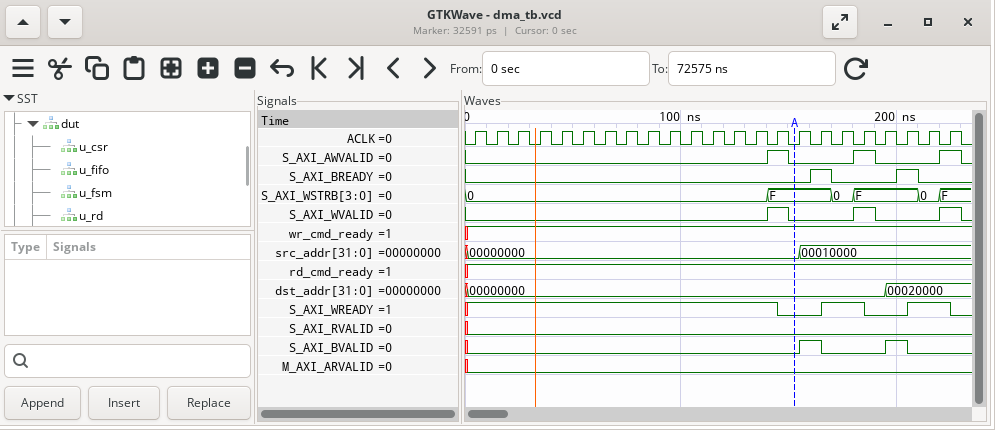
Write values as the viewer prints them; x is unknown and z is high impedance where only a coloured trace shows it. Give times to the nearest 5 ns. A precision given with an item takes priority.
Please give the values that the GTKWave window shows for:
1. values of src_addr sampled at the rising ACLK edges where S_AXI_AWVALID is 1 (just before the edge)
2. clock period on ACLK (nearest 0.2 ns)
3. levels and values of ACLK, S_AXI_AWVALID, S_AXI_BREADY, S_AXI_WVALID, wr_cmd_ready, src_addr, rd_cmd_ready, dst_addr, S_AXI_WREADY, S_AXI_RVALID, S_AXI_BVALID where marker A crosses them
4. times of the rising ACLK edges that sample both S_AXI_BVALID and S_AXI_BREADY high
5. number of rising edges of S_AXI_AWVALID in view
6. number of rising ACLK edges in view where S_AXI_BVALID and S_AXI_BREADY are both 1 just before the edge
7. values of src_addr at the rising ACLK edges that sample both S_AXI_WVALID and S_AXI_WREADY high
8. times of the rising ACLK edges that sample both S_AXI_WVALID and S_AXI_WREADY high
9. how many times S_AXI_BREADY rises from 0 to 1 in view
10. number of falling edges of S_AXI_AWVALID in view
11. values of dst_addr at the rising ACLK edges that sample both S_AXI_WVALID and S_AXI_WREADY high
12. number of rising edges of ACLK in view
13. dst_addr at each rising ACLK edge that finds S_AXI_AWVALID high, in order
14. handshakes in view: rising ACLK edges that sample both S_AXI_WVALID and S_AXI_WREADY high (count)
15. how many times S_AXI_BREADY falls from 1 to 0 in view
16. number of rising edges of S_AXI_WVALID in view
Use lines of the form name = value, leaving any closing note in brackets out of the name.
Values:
values of src_addr sampled at the rising ACLK edges where S_AXI_AWVALID is 1 = 00000000, 00010000, 00010000
clock period on ACLK = 10 ns
levels and values of ACLK, S_AXI_AWVALID, S_AXI_BREADY, S_AXI_WVALID, wr_cmd_ready, src_addr, rd_cmd_ready, dst_addr, S_AXI_WREADY, S_AXI_RVALID, S_AXI_BVALID where marker A crosses them = ACLK=0, S_AXI_AWVALID=0, S_AXI_BREADY=0, S_AXI_WVALID=0, wr_cmd_ready=1, src_addr=00000000, rd_cmd_ready=1, dst_addr=00000000, S_AXI_WREADY=0, S_AXI_RVALID=0, S_AXI_BVALID=0
times of the rising ACLK edges that sample both S_AXI_BVALID and S_AXI_BREADY high = 165 ns, 205 ns
number of rising edges of S_AXI_AWVALID in view = 3
number of rising ACLK edges in view where S_AXI_BVALID and S_AXI_BREADY are both 1 just before the edge = 2
values of src_addr at the rising ACLK edges that sample both S_AXI_WVALID and S_AXI_WREADY high = 00000000, 00010000, 00010000
times of the rising ACLK edges that sample both S_AXI_WVALID and S_AXI_WREADY high = 145 ns, 185 ns, 225 ns
how many times S_AXI_BREADY rises from 0 to 1 in view = 2
number of falling edges of S_AXI_AWVALID in view = 3
values of dst_addr at the rising ACLK edges that sample both S_AXI_WVALID and S_AXI_WREADY high = 00000000, 00000000, 00020000
number of rising edges of ACLK in view = 23
dst_addr at each rising ACLK edge that finds S_AXI_AWVALID high, in order = 00000000, 00000000, 00020000
handshakes in view: rising ACLK edges that sample both S_AXI_WVALID and S_AXI_WREADY high = 3
how many times S_AXI_BREADY falls from 1 to 0 in view = 2
number of rising edges of S_AXI_WVALID in view = 3
